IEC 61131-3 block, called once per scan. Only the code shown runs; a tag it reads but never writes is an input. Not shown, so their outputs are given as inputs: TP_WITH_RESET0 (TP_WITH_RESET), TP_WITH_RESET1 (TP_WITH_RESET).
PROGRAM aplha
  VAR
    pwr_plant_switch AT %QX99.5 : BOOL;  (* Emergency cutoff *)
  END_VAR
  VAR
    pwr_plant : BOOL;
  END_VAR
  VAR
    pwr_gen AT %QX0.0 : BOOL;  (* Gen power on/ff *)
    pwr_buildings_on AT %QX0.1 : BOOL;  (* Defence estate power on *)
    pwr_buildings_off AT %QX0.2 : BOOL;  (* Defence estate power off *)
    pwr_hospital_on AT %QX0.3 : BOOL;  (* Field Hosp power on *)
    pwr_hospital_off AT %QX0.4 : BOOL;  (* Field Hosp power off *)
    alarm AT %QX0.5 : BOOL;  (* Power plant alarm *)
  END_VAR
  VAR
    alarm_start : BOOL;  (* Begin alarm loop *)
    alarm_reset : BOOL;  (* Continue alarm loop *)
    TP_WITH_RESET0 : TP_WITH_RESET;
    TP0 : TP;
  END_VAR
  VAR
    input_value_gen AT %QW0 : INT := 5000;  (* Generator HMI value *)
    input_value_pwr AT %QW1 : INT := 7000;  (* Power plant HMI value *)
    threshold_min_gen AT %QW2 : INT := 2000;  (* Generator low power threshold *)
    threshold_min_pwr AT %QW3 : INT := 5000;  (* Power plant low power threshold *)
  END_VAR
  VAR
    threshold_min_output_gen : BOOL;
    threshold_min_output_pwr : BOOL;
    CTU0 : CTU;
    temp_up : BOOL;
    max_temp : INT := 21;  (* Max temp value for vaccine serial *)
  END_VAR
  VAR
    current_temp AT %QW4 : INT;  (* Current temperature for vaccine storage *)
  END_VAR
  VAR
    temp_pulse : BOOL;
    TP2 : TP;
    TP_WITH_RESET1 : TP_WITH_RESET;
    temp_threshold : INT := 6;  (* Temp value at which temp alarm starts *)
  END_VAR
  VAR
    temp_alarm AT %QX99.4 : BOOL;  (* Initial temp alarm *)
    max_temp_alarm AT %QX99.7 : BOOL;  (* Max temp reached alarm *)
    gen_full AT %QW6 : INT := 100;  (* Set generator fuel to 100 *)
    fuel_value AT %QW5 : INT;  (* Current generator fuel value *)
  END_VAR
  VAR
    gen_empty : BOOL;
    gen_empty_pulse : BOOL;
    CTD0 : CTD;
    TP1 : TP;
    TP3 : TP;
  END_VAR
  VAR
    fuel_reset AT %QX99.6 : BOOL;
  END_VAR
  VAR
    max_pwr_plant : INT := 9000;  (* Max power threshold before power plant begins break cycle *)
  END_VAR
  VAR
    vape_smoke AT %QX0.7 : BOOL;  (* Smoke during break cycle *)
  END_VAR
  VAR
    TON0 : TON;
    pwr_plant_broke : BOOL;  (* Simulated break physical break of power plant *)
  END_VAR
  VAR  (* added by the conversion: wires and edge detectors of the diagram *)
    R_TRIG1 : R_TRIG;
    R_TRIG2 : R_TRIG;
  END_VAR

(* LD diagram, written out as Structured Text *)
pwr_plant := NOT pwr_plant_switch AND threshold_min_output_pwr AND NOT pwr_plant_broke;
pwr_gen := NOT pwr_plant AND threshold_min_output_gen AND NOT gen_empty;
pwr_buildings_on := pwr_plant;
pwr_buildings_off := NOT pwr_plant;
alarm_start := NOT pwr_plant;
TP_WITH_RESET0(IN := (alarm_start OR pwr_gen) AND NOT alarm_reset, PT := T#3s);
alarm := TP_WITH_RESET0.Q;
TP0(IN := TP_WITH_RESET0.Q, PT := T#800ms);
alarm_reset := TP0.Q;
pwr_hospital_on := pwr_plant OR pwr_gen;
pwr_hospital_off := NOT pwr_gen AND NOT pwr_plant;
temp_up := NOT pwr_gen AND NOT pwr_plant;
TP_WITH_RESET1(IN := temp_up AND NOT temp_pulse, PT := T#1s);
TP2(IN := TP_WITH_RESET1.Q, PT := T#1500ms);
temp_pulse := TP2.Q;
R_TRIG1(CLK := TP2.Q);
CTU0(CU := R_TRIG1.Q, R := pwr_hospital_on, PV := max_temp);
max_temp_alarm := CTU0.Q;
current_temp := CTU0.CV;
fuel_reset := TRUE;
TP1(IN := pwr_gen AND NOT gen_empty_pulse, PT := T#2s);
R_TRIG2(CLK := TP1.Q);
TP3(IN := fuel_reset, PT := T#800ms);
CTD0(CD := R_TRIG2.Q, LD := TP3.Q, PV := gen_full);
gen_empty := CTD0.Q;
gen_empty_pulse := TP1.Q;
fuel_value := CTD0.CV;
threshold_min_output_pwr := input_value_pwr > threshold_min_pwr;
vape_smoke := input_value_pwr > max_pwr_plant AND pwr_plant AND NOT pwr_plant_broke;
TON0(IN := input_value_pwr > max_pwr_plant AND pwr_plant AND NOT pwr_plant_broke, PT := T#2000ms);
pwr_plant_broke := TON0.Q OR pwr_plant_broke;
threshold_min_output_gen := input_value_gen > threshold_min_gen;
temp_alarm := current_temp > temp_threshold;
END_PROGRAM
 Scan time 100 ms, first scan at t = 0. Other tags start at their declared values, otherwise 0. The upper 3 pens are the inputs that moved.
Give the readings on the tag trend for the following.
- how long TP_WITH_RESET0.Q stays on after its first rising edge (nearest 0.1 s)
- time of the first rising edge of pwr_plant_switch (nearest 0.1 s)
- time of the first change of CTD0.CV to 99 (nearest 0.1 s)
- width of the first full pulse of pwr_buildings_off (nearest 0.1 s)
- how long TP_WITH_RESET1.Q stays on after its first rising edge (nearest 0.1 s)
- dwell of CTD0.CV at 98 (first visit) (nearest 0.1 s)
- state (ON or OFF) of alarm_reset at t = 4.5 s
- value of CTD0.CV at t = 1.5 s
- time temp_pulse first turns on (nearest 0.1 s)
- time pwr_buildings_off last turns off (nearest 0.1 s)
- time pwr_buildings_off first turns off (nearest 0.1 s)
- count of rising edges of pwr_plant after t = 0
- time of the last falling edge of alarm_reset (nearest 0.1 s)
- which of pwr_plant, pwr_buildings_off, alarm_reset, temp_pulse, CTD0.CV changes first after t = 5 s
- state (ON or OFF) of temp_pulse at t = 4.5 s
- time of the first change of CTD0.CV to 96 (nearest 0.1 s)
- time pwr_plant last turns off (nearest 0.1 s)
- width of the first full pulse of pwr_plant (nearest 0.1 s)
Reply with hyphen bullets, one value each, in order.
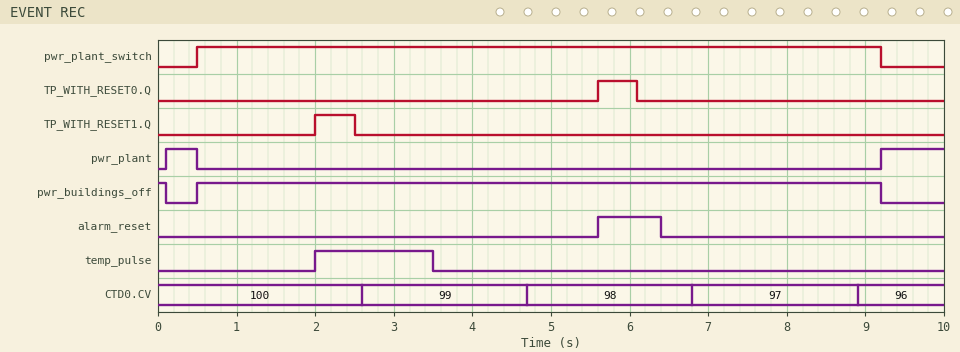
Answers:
- 0.5 s
- 0.5 s
- 2.6 s
- 8.7 s
- 0.5 s
- 2.1 s
- OFF
- 100
- 2.0 s
- 9.2 s
- 0.1 s
- 2
- 6.4 s
- alarm_reset
- OFF
- 8.9 s
- 0.5 s
- 0.4 s
